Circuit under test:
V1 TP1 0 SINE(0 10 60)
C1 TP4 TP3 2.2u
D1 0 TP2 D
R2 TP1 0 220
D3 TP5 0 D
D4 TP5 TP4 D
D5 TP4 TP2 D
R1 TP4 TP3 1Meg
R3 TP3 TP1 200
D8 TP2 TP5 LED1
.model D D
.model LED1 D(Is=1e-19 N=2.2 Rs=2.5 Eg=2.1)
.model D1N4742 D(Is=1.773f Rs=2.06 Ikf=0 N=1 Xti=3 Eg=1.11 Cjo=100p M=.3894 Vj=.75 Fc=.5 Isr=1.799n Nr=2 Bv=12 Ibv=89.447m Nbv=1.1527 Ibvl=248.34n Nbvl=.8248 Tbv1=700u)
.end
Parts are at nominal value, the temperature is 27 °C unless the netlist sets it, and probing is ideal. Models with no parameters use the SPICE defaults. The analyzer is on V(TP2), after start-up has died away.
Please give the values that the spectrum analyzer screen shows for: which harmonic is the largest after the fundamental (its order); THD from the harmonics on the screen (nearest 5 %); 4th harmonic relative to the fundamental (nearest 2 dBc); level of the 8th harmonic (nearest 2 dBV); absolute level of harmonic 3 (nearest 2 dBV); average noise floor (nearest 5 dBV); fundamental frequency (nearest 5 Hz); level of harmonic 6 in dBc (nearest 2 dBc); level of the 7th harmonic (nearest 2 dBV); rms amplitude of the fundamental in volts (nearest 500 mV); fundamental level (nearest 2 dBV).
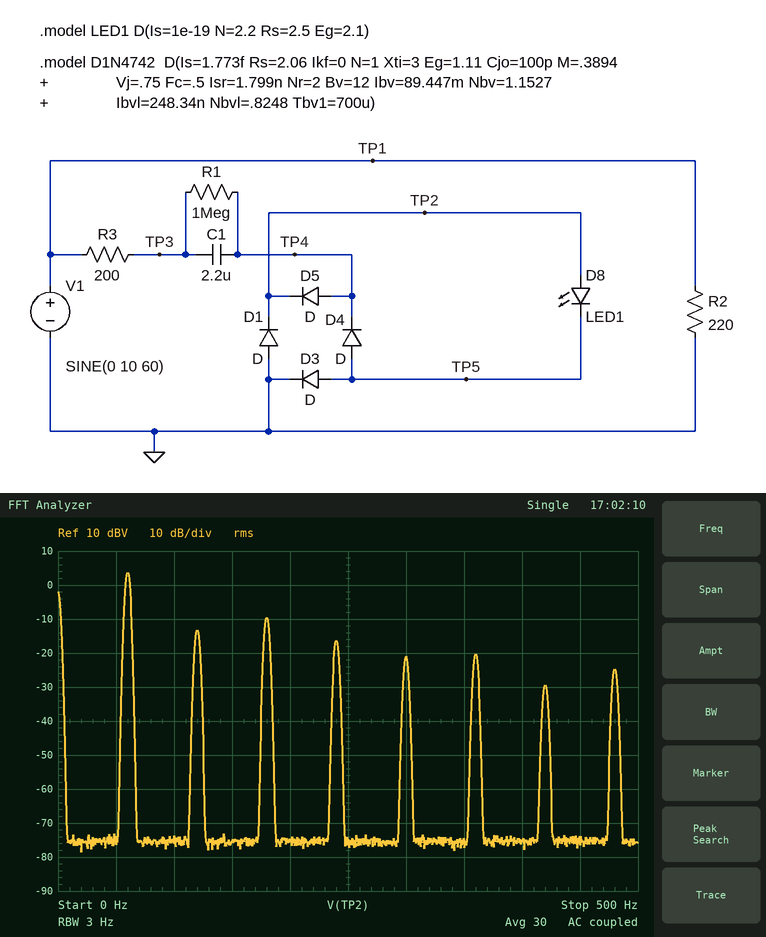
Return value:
3
30 %
-20 dBc
-24 dBV
-10 dBV
-75 dBV
60 Hz
-24 dBc
-30 dBV
1.5 V
4 dBV
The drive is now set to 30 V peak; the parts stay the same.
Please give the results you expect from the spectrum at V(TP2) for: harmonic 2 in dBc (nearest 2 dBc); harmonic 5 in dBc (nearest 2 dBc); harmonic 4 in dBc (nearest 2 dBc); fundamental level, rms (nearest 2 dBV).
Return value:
-22 dBc
-18 dBc
-24 dBc
4 dBV
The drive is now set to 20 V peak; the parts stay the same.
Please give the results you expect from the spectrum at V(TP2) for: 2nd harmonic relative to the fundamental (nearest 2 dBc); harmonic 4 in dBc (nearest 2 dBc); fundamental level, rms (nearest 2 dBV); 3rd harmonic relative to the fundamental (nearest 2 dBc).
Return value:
-20 dBc
-22 dBc
4 dBV
-12 dBc
